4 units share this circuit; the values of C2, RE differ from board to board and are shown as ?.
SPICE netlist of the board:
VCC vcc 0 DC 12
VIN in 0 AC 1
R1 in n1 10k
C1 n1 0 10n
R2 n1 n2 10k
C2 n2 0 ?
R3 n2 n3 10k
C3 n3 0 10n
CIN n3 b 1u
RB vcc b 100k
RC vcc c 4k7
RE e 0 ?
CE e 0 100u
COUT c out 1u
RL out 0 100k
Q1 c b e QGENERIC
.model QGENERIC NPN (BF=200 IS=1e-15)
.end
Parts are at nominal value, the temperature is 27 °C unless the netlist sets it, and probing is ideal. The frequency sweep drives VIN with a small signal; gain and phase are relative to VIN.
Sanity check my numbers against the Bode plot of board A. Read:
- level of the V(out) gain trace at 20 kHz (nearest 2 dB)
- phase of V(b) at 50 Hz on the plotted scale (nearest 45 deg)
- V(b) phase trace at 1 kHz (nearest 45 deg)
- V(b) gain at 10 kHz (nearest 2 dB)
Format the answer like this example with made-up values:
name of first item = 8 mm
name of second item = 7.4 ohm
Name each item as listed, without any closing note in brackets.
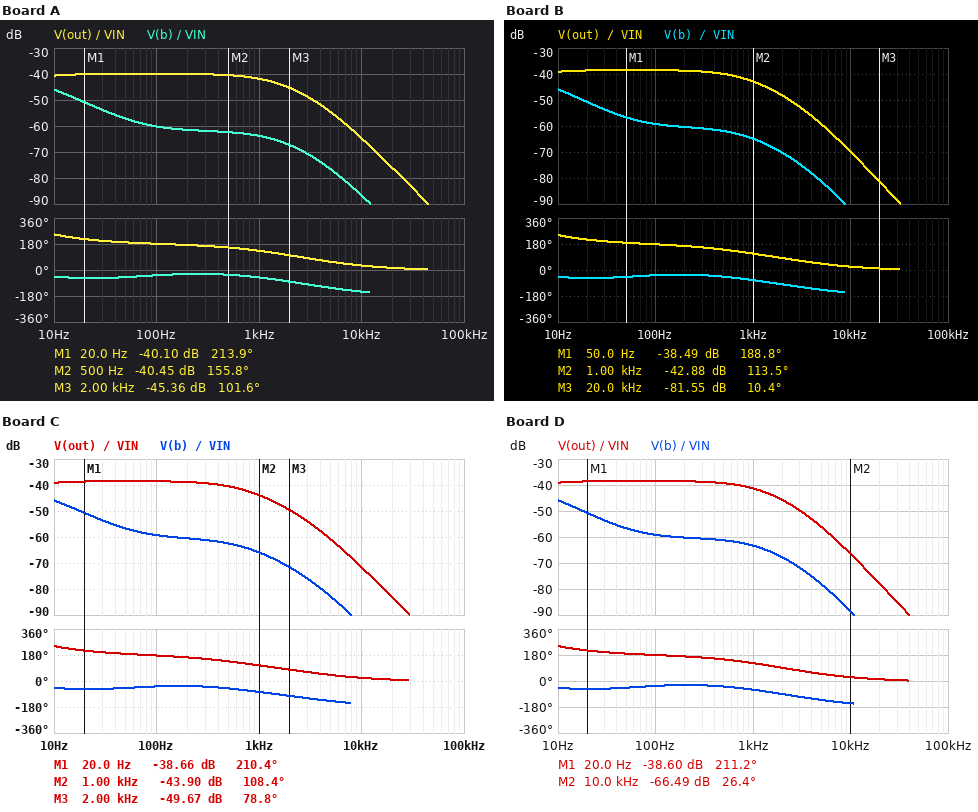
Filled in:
level of the V(out) gain trace at 20 kHz = -76 dB
phase of V(b) at 50 Hz on the plotted scale = -45 deg
V(b) phase trace at 1 kHz = -45 deg
V(b) gain at 10 kHz = -86 dB
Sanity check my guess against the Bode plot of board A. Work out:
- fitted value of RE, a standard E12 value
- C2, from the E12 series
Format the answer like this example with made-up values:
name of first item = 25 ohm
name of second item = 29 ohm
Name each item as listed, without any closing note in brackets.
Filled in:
fitted value of RE, a standard E12 value = 1.2 kΩ
C2, from the E12 series = 12 nF
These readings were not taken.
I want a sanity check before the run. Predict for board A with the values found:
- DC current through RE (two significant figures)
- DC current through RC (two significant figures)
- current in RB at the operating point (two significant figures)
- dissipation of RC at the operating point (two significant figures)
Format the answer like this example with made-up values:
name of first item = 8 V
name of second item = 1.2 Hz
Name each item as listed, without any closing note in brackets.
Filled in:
DC current through RE = 2.1 mA
DC current through RC = 2.0 mA
current in RB at the operating point = 88 µA
dissipation of RC at the operating point = 19 mW
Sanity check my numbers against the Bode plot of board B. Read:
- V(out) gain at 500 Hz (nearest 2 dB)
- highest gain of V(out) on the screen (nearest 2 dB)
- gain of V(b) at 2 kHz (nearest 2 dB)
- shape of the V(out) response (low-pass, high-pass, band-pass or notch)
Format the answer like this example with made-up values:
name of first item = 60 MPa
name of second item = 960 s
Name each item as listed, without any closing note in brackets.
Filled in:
V(out) gain at 500 Hz = -40 dB
highest gain of V(out) on the screen = -38 dB
gain of V(b) at 2 kHz = -70 dB
shape of the V(out) response = low-pass
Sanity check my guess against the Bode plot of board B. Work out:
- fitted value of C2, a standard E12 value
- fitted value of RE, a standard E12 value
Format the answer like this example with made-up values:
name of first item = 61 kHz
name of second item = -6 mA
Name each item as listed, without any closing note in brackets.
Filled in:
fitted value of C2, a standard E12 value = 27 nF
fitted value of RE, a standard E12 value = 2.2 kΩ
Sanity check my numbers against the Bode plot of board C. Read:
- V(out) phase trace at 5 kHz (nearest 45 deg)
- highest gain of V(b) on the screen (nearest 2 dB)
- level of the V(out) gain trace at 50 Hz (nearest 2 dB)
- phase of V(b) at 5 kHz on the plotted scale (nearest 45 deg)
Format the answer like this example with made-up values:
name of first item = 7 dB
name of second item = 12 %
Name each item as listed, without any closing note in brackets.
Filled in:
V(out) phase trace at 5 kHz = 45 deg
highest gain of V(b) on the screen = -46 dB
level of the V(out) gain trace at 50 Hz = -38 dB
phase of V(b) at 5 kHz on the plotted scale = -135 deg
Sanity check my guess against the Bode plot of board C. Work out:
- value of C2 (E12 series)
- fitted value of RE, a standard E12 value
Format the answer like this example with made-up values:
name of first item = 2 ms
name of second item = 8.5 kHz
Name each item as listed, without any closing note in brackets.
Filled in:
value of C2 = 33 nF
fitted value of RE, a standard E12 value = 2.2 kΩ
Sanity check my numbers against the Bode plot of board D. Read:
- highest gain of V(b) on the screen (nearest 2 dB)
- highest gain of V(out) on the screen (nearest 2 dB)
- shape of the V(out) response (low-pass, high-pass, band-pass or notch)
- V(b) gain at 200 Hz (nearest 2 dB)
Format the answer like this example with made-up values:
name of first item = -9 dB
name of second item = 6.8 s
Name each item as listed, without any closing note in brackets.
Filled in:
highest gain of V(b) on the screen = -46 dB
highest gain of V(out) on the screen = -38 dB
shape of the V(out) response = low-pass
V(b) gain at 200 Hz = -60 dB
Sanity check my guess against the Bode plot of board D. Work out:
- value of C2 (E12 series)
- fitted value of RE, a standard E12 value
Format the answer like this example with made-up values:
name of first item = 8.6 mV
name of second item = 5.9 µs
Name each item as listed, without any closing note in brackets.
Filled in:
value of C2 = 18 nF
fitted value of RE, a standard E12 value = 2.2 kΩ
